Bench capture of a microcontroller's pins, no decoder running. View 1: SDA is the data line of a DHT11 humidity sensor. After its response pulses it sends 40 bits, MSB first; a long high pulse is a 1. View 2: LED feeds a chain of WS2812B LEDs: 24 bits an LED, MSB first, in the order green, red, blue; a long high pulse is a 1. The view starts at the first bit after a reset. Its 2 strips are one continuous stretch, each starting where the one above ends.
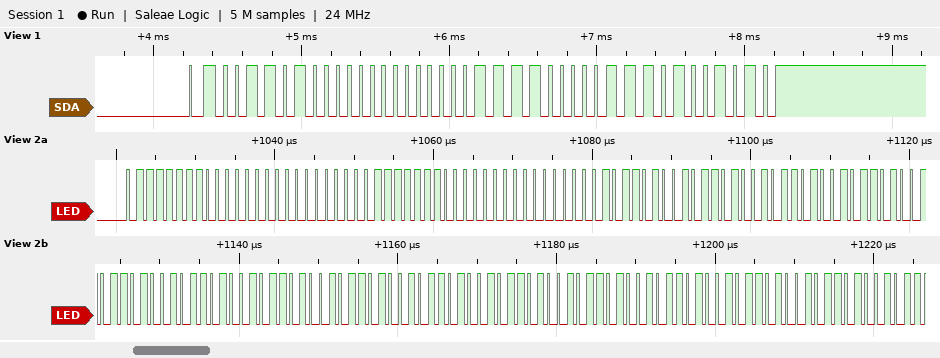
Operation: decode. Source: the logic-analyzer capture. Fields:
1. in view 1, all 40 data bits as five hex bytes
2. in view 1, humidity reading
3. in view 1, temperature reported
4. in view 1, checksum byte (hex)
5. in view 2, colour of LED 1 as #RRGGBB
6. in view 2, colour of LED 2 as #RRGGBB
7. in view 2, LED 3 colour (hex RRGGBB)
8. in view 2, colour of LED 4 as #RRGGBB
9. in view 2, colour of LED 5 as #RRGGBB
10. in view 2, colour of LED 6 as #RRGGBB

34 00 0F 07 4A
52 %
15.7 °C
0x4A
#007F00
#007F00
#B4B4B4
#B4B4B4
#B4B4B4
#B4B4B4
